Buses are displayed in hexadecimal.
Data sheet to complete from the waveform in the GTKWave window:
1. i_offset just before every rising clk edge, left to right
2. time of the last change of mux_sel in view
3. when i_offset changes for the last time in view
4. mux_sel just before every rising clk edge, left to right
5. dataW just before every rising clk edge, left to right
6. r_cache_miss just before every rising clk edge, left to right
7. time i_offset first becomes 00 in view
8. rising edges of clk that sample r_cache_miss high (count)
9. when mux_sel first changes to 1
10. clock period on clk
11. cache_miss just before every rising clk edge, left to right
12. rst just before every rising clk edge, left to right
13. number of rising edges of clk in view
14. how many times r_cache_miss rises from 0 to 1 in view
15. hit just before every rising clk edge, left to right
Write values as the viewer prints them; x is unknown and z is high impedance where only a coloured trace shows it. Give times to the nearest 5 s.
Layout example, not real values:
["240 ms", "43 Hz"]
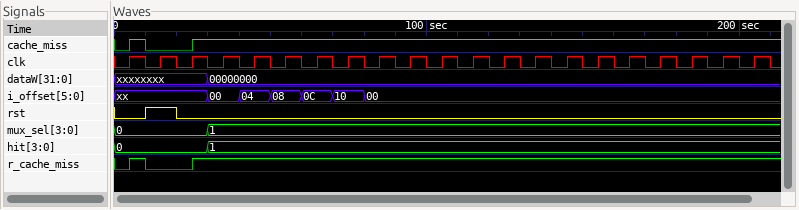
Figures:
["xx, xx, xx, 00, 04, 08, 0C, 10, 00, 00, 00, 00, 00, 00, 00, 00, 00, 00, 00, 00, 00", "30 s", "80 s", "0, 0, 0, 1, 1, 1, 1, 1, 1, 1, 1, 1, 1, 1, 1, 1, 1, 1, 1, 1, 1", "xxxxxxxx, xxxxxxxx, xxxxxxxx, 00000000, 00000000, 00000000, 00000000, 00000000, 00000000, 00000000, 00000000, 00000000, 00000000, 00000000, 00000000, 00000000, 00000000, 00000000, 00000000, 00000000, 00000000", "0 0 0 1 1 1 1 1 1 1 1 1 1 1 1 1 1 1 1 1 1", "30 s", "18", "30 s", "10 s", "0 0 0 1 1 1 1 1 1 1 1 1 1 1 1 1 1 1 1 1 1", "0 1 0 0 0 0 0 0 0 0 0 0 0 0 0 0 0 0 0 0 0", "21", "2", "0, 0, 0, 1, 1, 1, 1, 1, 1, 1, 1, 1, 1, 1, 1, 1, 1, 1, 1, 1, 1"]
